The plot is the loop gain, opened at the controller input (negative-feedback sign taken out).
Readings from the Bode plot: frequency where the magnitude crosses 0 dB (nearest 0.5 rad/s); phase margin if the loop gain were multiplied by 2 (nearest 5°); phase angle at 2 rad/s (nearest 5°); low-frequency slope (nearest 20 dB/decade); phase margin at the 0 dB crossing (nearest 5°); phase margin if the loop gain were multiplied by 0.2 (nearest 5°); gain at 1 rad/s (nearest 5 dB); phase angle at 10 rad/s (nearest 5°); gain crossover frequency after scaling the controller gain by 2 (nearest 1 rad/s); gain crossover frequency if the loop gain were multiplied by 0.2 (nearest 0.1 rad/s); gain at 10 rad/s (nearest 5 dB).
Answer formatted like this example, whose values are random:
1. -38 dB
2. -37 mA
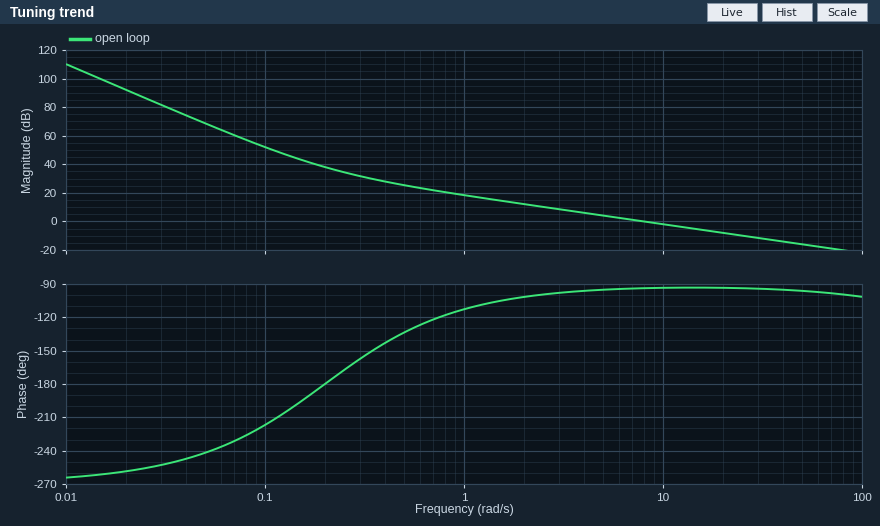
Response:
1. 8.0 rad/s
2. 85°
3. -100°
4. -60 dB/decade
5. 85°
6. 75°
7. 20 dB
8. -95°
9. 16 rad/s
10. 1.6 rad/s
11. 0 dB
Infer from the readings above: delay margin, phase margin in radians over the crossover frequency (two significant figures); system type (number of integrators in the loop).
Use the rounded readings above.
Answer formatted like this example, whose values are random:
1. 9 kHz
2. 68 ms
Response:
1. 0.19 s
2. 3
